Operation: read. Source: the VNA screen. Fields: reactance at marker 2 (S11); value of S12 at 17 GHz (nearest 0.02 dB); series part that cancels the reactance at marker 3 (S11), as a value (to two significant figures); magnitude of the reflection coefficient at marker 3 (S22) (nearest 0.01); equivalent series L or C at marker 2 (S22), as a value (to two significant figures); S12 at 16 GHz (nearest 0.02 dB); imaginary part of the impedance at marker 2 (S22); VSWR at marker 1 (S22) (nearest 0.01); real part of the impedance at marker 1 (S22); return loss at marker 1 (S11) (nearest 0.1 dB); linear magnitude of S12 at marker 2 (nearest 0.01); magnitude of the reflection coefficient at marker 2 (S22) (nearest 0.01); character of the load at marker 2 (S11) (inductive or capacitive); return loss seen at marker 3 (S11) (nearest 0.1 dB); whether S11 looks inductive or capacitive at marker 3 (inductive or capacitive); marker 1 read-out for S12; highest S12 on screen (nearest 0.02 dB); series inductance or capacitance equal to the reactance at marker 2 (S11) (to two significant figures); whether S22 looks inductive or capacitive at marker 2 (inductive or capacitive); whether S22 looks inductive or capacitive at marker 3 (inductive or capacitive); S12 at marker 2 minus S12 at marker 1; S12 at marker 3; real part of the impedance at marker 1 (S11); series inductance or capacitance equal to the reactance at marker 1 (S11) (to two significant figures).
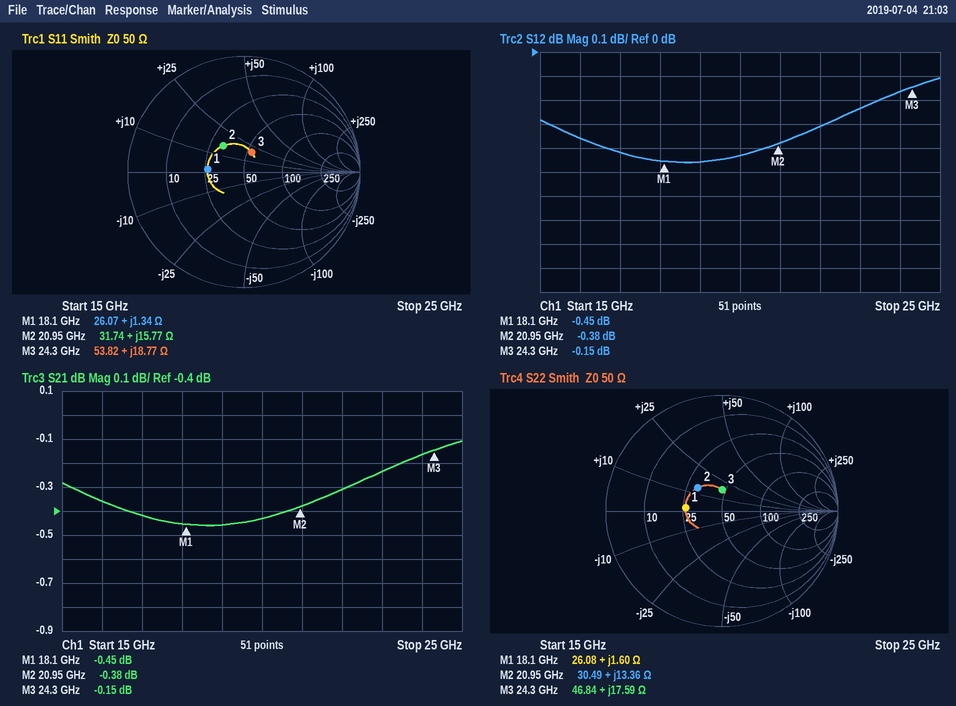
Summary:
+15.77 Ω
-0.42 dB
350 fF
0.18
100 pH
-0.36 dB
+13.36 Ω
1.92
26.08 Ω
10.0 dB
0.96
0.29
inductive
14.8 dB
inductive
-0.45 dB
-0.10 dB
120 pH
inductive
inductive
0.07 dB
-0.15 dB
26.07 Ω
12 pH
